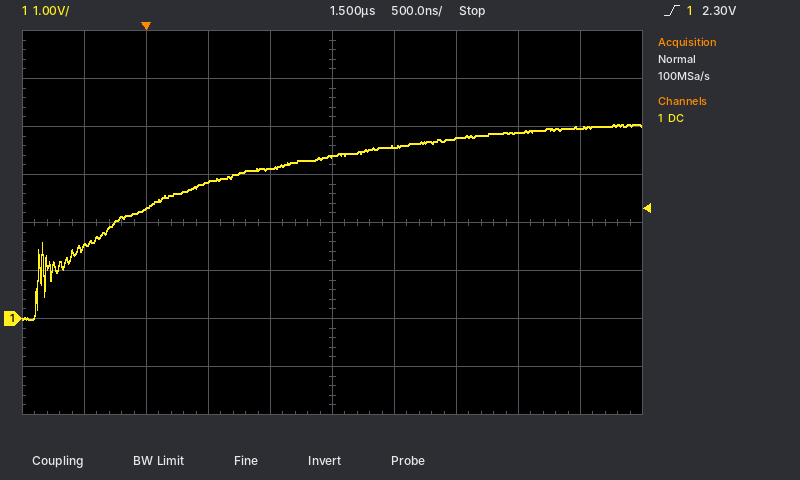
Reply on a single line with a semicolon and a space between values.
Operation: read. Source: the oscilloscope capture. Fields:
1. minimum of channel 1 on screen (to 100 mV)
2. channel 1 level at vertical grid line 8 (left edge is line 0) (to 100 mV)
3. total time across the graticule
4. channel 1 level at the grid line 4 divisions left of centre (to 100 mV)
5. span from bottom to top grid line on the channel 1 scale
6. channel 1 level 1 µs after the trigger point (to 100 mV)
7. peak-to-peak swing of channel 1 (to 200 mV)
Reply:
0.0 V; 3.9 V; 5 µs; 1.5 V; 8 V; 3.1 V; 4.0 V
